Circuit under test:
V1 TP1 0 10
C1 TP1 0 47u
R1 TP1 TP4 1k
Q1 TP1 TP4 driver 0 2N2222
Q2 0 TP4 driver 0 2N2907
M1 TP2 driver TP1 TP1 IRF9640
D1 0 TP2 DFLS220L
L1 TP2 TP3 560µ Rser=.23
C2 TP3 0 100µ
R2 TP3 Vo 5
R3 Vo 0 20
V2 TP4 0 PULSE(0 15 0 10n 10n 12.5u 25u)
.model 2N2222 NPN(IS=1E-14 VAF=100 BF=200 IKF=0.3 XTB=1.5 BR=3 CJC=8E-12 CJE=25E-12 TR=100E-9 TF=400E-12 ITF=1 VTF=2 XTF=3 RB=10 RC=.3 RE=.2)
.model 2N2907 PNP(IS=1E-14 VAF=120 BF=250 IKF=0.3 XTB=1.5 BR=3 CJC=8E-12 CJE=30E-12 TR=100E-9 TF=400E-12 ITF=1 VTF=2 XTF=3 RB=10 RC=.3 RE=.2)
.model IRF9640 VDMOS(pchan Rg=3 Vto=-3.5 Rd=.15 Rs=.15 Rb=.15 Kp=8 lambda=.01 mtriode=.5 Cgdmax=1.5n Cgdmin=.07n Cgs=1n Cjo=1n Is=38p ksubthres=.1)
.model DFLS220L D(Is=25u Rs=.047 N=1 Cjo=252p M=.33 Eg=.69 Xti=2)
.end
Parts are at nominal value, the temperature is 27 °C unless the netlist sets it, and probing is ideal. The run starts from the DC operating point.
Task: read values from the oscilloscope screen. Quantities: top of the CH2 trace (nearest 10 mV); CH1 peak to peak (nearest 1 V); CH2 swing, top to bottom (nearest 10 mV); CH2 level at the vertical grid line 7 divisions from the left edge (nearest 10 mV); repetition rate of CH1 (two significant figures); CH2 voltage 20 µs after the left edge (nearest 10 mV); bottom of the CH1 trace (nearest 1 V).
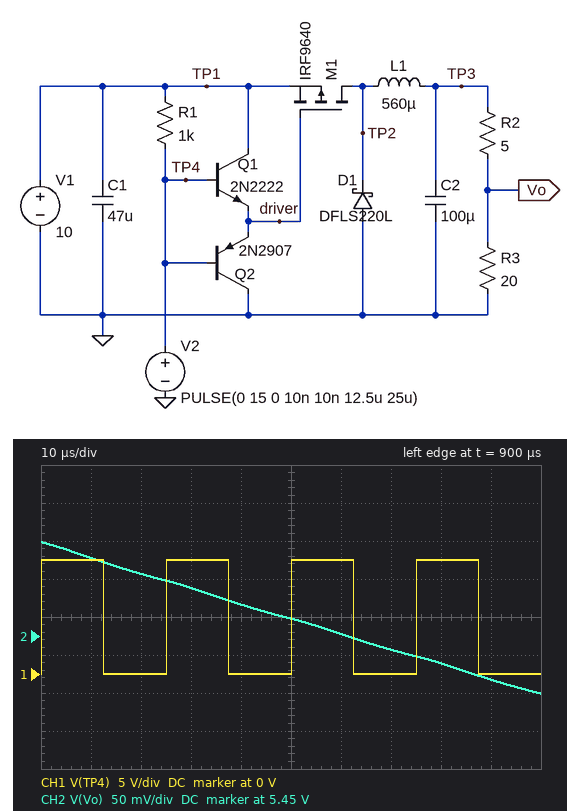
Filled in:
5.57 V
15 V
200 mV
5.43 V
40 kHz
5.53 V
0 V
